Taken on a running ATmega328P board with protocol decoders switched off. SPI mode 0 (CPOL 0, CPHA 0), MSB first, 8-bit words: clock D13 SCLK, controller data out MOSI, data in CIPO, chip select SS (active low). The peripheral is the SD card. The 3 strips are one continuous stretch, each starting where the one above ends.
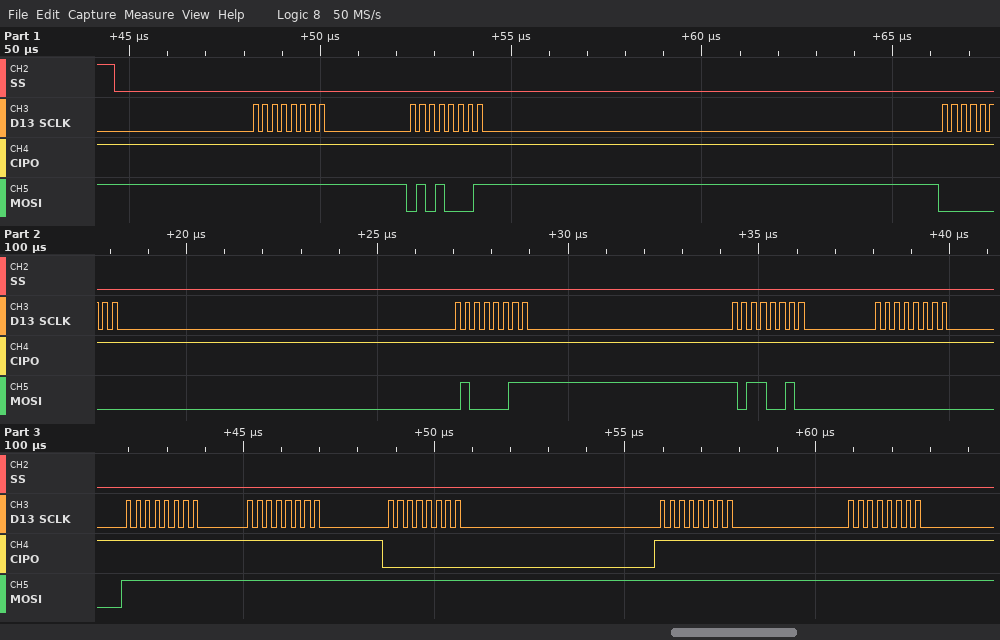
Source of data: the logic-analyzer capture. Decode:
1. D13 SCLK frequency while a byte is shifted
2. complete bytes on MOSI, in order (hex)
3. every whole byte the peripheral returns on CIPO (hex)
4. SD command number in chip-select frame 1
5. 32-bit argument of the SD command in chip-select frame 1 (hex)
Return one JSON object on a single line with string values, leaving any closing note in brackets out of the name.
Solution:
{"D13 SCLK frequency while a byte is shifted": "4 MHz", "complete bytes on MOSI, in order": "0xFF 0x51 0x00 0x43 0xB2 0x00 0xFF 0xFF 0xFF 0xFF 0xFF", "every whole byte the peripheral returns on CIPO": "0xFF 0xFF 0xFF 0xFF 0xFF 0xFF 0xFF 0xFF 0x00 0xFF 0xFF", "SD command number in chip-select frame 1": "CMD17", "32-bit argument of the SD command in chip-select frame 1": "0x0043B200"}
